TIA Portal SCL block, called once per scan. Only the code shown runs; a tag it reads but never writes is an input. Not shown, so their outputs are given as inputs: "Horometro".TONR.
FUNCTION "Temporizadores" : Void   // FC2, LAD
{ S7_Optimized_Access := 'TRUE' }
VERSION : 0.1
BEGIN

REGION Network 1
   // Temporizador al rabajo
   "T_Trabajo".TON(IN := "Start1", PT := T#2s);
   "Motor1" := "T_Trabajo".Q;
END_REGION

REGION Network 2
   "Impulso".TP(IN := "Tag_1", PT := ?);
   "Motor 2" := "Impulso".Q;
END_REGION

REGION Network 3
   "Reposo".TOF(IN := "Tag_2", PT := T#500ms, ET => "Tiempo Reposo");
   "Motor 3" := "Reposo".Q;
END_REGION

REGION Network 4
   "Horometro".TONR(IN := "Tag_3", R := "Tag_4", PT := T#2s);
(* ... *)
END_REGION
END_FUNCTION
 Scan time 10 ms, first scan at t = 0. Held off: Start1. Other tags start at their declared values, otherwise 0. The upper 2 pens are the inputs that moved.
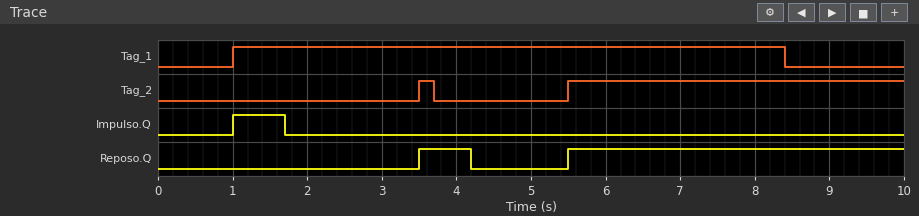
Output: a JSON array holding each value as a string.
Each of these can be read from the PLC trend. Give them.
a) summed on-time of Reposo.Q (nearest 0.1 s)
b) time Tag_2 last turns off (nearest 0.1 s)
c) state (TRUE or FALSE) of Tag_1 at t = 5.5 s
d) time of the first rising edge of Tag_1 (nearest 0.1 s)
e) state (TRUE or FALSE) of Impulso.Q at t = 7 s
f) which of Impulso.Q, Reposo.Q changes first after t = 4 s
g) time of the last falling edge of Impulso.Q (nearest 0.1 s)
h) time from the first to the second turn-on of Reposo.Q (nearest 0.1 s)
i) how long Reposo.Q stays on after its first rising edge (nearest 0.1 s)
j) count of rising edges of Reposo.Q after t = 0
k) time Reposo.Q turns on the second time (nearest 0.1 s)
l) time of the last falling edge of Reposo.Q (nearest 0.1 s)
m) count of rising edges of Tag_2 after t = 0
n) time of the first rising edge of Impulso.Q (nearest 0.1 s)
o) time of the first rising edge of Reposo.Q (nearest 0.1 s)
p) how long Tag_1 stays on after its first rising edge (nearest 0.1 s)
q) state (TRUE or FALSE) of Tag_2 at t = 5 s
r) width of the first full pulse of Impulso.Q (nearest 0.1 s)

["5.2 s", "3.7 s", "TRUE", "1.0 s", "FALSE", "Reposo.Q", "1.7 s", "2.0 s", "0.7 s", "2", "5.5 s", "4.2 s", "2", "1.0 s", "3.5 s", "7.4 s", "FALSE", "0.7 s"]
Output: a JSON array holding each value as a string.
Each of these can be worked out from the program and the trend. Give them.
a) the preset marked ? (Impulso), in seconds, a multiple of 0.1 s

["0.7 s"]
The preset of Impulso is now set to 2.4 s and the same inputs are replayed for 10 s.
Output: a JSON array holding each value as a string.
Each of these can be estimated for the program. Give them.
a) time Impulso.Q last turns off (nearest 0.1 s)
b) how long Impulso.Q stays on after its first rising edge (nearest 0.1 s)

["3.4 s", "2.4 s"]
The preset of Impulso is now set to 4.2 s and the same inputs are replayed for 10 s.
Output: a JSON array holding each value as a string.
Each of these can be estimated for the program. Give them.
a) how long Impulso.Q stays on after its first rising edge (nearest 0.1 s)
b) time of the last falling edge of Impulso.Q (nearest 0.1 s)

["4.2 s", "5.2 s"]
